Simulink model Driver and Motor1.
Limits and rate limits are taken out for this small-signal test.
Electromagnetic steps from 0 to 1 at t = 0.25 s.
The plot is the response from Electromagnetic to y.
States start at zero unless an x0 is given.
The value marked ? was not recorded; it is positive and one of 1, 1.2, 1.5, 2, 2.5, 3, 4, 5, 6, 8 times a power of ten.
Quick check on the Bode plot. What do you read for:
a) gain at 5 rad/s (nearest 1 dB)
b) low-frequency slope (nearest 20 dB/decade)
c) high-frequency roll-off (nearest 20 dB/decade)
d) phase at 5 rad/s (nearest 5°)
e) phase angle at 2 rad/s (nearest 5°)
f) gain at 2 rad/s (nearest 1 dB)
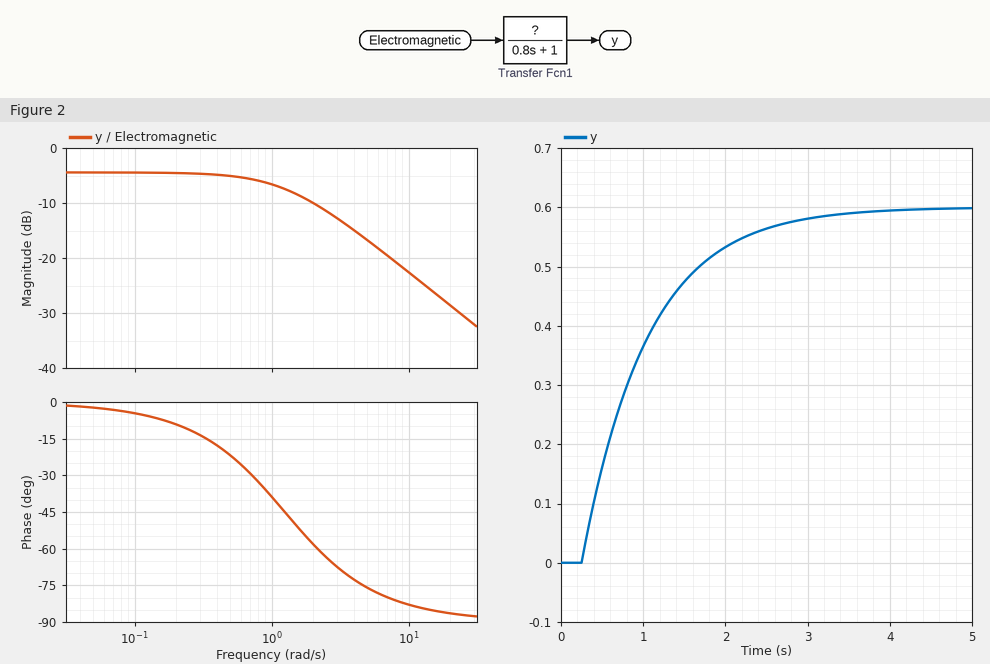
-17 dB
0 dB/decade
-20 dB/decade
-75°
-60°
-10 dB
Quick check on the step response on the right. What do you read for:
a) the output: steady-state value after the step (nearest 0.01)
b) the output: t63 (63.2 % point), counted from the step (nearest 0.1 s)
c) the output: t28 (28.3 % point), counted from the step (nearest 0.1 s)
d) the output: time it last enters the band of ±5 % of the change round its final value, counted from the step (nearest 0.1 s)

0.60
0.8 s
0.3 s
2.4 s
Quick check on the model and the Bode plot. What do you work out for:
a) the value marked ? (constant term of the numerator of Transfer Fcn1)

0.6
